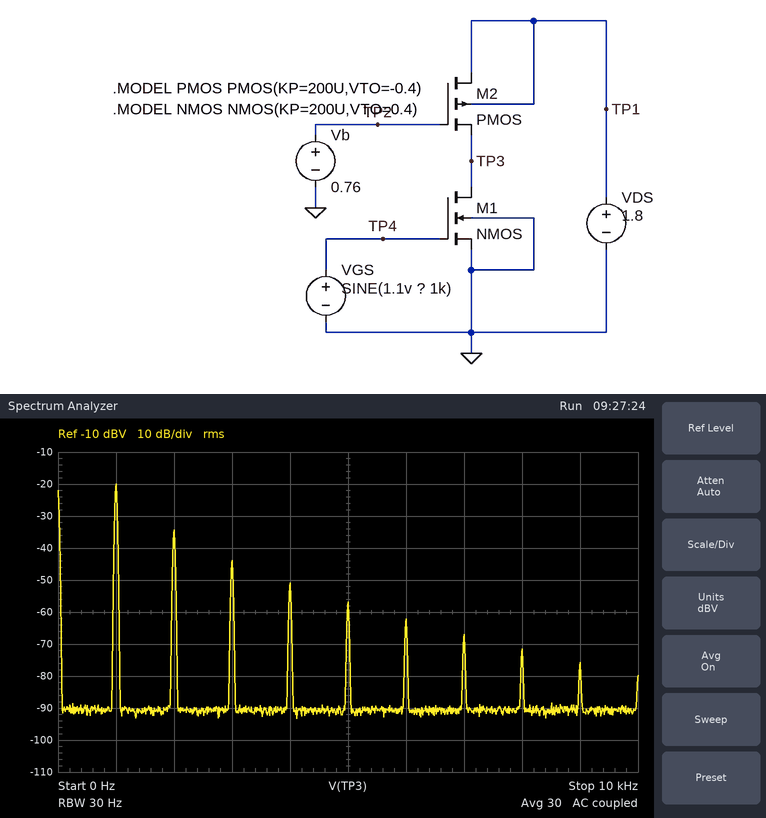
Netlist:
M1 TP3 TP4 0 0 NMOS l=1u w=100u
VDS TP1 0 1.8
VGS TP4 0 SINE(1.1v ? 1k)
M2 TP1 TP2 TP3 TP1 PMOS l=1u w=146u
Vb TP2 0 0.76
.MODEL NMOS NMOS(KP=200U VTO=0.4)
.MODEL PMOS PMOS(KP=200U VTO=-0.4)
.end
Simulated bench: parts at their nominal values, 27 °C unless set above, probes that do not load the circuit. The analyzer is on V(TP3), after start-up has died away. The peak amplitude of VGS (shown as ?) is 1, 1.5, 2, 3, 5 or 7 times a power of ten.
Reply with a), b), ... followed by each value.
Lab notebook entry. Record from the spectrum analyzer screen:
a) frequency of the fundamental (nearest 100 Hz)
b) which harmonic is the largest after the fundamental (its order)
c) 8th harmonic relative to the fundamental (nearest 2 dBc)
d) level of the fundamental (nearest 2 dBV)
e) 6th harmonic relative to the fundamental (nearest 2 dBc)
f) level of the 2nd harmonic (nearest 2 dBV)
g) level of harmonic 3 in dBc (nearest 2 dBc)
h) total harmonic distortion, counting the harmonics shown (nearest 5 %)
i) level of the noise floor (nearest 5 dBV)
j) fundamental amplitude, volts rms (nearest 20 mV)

a) 1.0 kHz
b) 2
c) -52 dBc
d) -20 dBV
e) -42 dBc
f) -34 dBV
g) -24 dBc
h) 20 %
i) -90 dBV
j) 100 mV
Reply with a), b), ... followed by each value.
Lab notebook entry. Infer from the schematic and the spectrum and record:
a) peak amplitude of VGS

a) 70 mV
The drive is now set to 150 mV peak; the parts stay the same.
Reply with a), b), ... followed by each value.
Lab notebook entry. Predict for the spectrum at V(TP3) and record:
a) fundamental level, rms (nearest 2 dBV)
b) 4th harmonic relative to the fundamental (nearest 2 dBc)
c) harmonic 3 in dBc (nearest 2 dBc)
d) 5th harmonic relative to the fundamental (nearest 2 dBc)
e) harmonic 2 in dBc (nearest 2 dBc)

a) -8 dBV
b) -16 dBc
c) -34 dBc
d) -20 dBc
e) -10 dBc
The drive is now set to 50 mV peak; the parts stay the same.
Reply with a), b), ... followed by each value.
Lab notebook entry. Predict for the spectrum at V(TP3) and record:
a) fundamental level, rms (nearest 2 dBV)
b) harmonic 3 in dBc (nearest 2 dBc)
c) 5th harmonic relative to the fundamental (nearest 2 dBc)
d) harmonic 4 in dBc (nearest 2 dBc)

a) -24 dBV
b) -34 dBc
c) -58 dBc
d) -46 dBc
